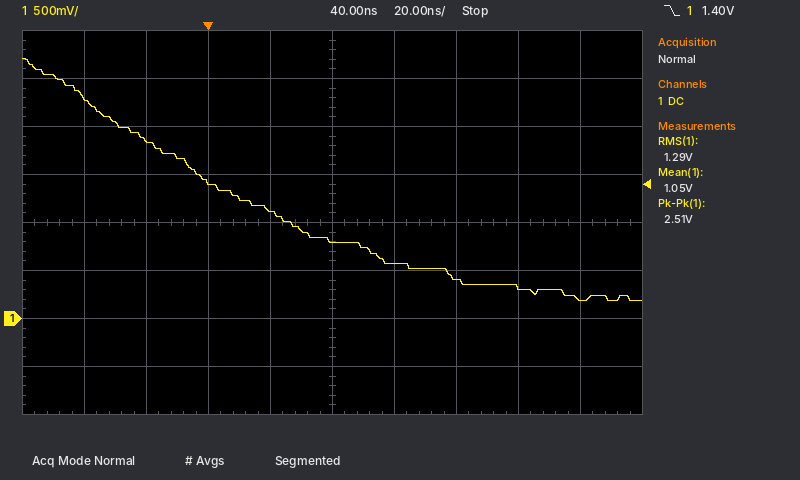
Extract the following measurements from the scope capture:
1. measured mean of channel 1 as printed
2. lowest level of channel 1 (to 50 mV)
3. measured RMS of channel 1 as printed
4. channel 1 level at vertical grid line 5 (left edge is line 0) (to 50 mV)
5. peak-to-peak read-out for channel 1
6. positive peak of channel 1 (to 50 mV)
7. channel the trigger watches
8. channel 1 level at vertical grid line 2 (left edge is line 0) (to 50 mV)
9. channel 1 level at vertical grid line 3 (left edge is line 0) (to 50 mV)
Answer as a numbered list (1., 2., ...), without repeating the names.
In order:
1. 1.05 V
2. 200 mV
3. 1.29 V
4. 800 mV
5. 2.51 V
6. 2.70 V
7. channel 1
8. 1.85 V
9. 1.40 V
